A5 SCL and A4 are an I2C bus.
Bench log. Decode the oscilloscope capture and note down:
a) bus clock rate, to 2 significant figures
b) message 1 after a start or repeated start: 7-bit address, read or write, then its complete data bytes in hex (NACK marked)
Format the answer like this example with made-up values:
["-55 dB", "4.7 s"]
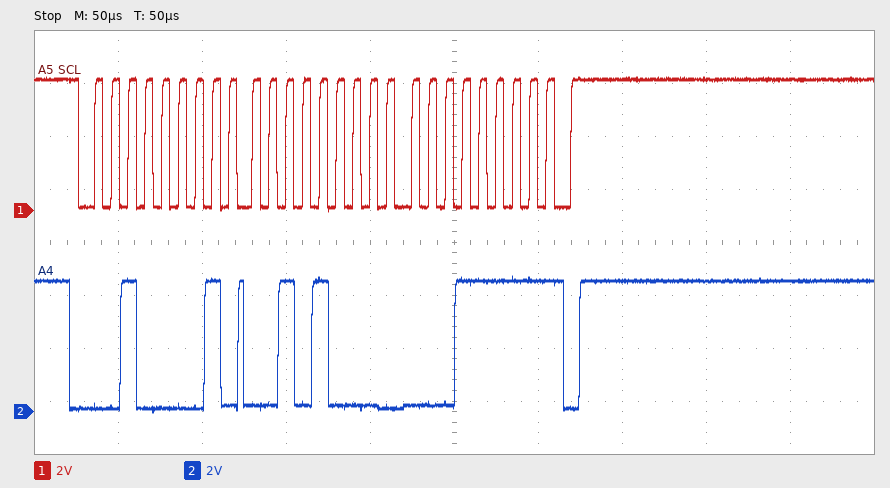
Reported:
["100 kHz", "0x10 read: 28 1F NACK"]
